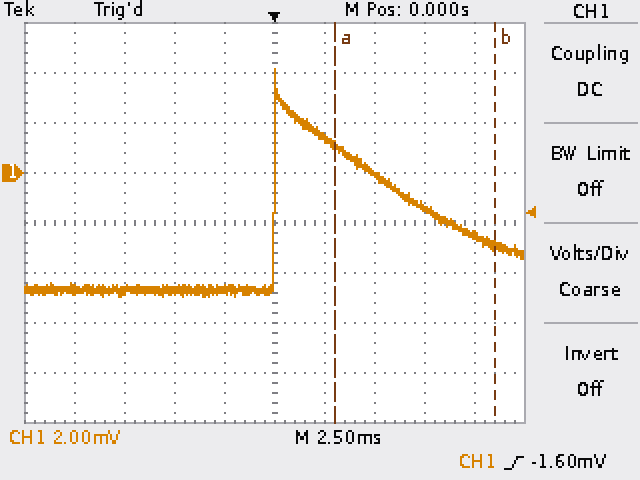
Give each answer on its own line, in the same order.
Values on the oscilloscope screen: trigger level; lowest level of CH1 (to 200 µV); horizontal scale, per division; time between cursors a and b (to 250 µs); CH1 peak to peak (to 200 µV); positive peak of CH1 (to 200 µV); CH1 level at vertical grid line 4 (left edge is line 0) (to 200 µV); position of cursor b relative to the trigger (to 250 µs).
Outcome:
-1.60 mV
-5.0 mV
2.5 ms
8.00 ms
9.2 mV
4.2 mV
-4.6 mV
+11.00 ms
